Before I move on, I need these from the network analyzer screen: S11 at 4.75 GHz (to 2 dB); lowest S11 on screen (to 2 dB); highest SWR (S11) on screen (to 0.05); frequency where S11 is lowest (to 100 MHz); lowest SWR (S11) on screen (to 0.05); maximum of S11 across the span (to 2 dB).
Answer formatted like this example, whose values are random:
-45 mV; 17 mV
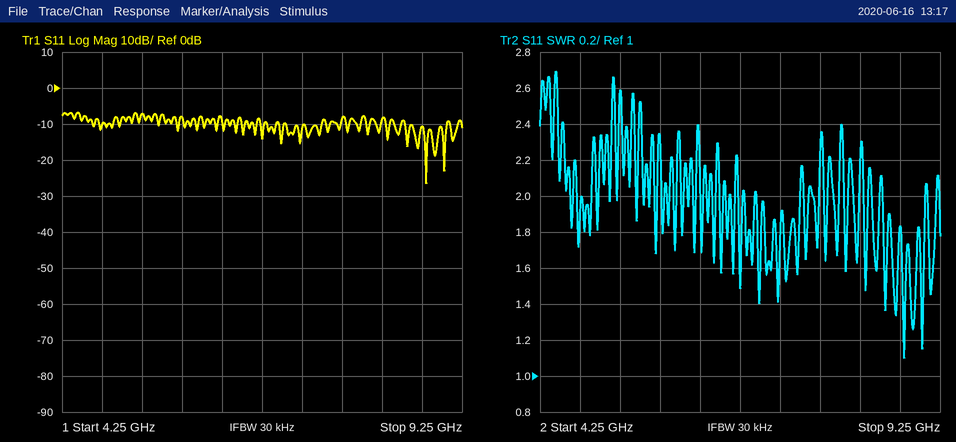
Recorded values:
-10 dB; -26 dB; 2.70; 8.8 GHz; 1.10; -6 dB
